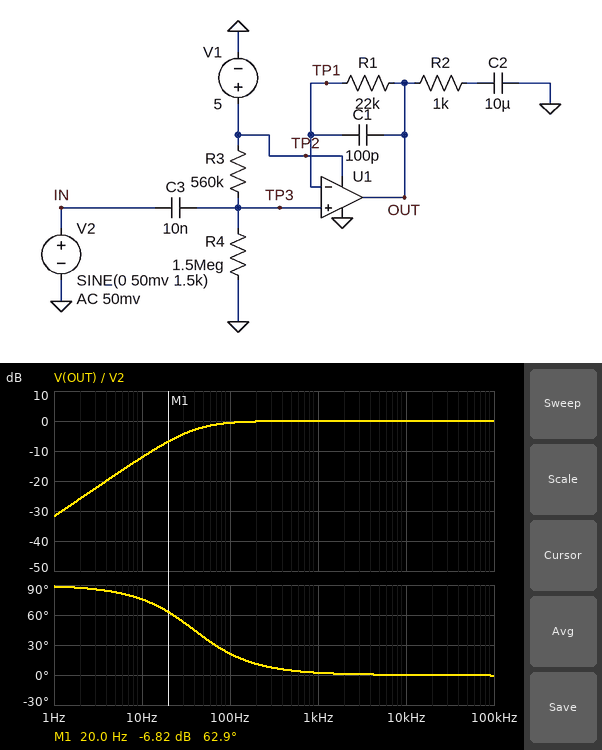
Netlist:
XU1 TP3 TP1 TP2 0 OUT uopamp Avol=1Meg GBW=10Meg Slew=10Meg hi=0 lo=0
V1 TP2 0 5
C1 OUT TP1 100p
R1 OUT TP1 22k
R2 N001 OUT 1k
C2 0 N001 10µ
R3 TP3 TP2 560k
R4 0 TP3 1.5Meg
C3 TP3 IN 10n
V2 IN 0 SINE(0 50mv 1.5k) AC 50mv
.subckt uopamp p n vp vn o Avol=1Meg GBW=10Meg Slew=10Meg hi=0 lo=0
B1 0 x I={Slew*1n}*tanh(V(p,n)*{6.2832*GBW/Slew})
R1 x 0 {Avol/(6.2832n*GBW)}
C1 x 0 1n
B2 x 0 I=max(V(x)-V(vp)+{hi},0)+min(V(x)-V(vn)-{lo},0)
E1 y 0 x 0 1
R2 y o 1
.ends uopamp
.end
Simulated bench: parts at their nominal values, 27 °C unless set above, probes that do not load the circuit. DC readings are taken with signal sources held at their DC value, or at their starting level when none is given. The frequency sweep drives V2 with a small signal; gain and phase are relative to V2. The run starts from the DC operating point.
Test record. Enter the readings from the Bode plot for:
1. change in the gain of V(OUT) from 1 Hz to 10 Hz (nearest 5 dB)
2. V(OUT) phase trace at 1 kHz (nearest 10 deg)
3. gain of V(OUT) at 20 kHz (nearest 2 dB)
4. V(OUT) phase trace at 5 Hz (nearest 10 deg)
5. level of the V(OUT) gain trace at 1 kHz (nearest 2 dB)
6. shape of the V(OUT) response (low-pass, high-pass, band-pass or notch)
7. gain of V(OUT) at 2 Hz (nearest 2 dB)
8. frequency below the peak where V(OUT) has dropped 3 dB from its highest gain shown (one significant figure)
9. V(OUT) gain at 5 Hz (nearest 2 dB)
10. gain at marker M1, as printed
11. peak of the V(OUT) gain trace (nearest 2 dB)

20 dB
0 deg
0 dB
80 deg
0 dB
high-pass
-26 dB
40 Hz
-18 dB
-6.82 dB
0 dB
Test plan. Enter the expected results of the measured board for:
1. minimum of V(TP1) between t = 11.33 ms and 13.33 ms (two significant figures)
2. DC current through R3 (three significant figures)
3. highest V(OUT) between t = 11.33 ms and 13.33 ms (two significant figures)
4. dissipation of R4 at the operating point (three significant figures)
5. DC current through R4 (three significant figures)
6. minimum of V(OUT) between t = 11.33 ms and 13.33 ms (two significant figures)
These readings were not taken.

3.6 V
2.43 µA
3.7 V
8.84 µW
2.43 µA
3.6 V
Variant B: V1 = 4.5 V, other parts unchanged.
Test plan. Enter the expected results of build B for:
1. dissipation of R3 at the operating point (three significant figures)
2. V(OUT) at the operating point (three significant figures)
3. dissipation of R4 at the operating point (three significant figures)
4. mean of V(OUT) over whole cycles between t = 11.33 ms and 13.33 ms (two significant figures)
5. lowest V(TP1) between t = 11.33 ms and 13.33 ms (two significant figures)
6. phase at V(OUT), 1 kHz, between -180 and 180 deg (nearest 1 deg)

2.67 µW
3.28 V
7.16 µW
3.3 V
3.2 V
2 deg
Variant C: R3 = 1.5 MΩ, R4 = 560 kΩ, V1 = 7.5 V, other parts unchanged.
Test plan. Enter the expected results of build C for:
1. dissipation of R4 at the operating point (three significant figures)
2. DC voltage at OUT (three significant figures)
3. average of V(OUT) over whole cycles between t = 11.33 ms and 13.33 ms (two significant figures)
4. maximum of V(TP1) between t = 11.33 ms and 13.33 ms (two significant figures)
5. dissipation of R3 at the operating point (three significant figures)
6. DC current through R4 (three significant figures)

7.42 µW
2.04 V
2.0 V
2.1 V
19.9 µW
3.64 µA
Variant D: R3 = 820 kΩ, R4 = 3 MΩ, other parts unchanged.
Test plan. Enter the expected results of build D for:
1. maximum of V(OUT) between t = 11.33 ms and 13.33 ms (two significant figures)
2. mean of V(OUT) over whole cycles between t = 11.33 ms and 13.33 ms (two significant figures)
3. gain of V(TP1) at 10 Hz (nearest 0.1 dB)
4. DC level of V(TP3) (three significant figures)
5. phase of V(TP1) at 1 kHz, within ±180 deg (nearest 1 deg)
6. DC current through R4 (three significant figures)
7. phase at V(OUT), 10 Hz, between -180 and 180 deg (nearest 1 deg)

4.0 V
3.9 V
-8.5 dB
3.93 V
1 deg
1.31 µA
68 deg
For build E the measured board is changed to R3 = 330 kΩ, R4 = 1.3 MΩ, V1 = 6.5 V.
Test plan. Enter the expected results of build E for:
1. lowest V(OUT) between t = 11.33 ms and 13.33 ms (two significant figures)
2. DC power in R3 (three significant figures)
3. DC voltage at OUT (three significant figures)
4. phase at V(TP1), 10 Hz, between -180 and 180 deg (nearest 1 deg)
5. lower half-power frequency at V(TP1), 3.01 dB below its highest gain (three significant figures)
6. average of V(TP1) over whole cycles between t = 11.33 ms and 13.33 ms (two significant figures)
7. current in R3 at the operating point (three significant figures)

5.1 V
5.25 µW
5.18 V
81 deg
60.5 Hz
5.2 V
3.99 µA
